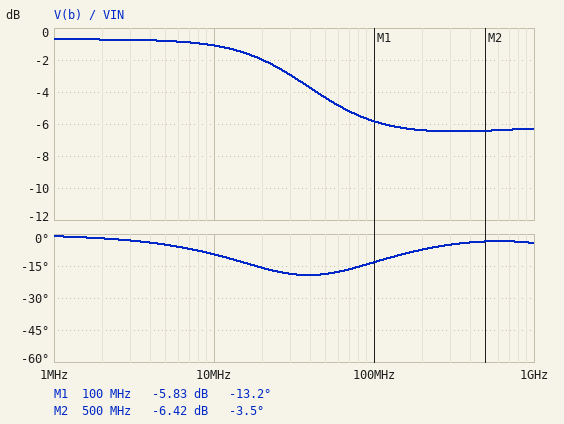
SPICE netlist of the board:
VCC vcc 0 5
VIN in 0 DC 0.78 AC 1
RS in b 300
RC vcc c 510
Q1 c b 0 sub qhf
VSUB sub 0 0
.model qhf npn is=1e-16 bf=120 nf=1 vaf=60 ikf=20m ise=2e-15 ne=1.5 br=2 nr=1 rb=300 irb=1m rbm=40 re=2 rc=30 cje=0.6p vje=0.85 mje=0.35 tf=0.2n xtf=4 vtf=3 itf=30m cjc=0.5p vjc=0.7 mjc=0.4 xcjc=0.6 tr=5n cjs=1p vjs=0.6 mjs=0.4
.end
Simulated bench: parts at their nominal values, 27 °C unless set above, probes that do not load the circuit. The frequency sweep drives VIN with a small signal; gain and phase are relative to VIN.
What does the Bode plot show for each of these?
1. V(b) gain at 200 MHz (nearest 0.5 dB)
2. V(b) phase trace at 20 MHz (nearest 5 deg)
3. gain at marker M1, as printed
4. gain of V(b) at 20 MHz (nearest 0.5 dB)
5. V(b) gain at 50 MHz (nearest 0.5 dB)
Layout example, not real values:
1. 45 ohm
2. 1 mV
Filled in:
1. -6.5 dB
2. -15 deg
3. -5.83 dB
4. -2.0 dB
5. -4.5 dB
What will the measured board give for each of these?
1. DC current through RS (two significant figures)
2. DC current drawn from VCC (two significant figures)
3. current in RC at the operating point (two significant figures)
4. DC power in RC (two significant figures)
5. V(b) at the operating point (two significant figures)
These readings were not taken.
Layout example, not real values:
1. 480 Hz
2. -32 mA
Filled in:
1. 8.8 µA
2. 960 µA
3. 960 µA
4. 470 µW
5. 780 mV
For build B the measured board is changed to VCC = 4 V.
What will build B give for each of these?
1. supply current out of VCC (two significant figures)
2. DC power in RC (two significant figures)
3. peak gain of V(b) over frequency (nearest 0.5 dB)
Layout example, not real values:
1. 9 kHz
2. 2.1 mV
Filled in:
1. 950 µA
2. 460 µW
3. -0.5 dB
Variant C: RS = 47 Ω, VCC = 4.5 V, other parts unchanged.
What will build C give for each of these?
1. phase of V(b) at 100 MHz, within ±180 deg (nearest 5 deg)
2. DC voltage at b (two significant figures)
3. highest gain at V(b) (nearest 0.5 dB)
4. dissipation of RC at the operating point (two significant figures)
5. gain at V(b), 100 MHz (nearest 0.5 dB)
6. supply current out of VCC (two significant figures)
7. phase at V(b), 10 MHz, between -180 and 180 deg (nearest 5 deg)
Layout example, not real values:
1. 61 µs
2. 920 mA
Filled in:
1. -5 deg
2. 780 mV
3. 0 dB
4. 530 µW
5. -1.0 dB
6. 1.0 mA
7. 0 deg
